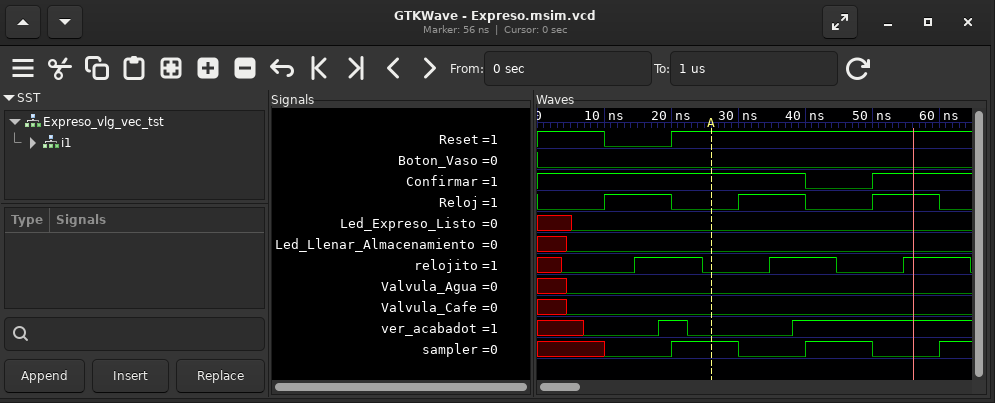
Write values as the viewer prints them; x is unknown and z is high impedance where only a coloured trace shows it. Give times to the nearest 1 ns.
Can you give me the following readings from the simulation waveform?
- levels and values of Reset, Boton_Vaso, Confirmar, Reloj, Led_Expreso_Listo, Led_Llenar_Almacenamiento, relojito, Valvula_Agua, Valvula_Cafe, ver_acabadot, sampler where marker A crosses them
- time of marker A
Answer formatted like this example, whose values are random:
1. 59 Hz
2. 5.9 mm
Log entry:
1. Reset=1, Boton_Vaso=0, Confirmar=1, Reloj=0, Led_Expreso_Listo=0, Led_Llenar_Almacenamiento=0, relojito=0, Valvula_Agua=0, Valvula_Cafe=0, ver_acabadot=0, sampler=1
2. 26 ns
